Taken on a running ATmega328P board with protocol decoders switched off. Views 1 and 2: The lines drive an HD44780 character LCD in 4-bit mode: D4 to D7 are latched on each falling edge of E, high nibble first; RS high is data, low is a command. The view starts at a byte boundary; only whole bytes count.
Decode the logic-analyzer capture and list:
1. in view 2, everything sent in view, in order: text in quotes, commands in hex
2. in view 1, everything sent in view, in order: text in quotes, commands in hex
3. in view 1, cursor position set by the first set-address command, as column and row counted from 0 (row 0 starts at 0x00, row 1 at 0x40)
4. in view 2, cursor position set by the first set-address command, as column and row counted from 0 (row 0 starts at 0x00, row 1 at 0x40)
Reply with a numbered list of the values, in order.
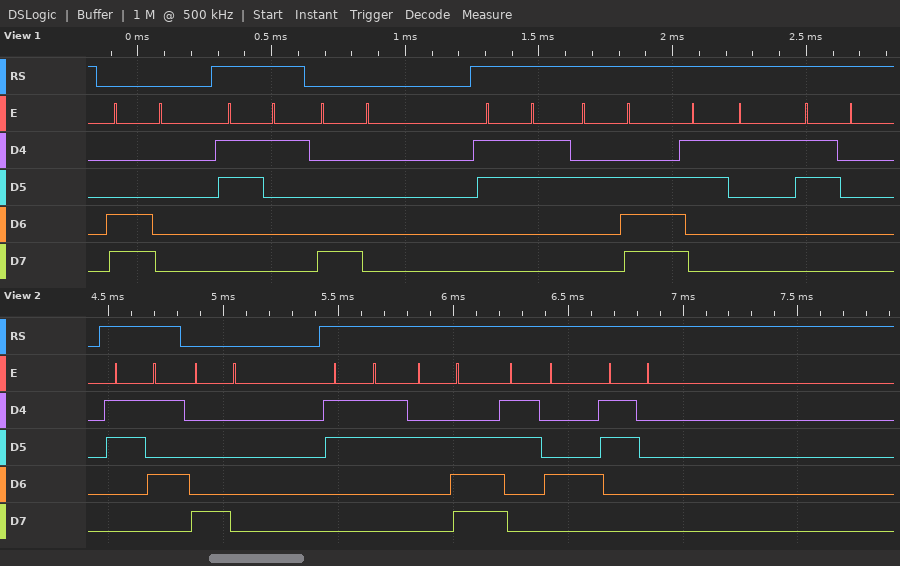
1. "5" 0x80 "3.40"
2. 0xC0 "1" 0x80 "3.10"
3. column 0, row 1
4. column 0, row 0
